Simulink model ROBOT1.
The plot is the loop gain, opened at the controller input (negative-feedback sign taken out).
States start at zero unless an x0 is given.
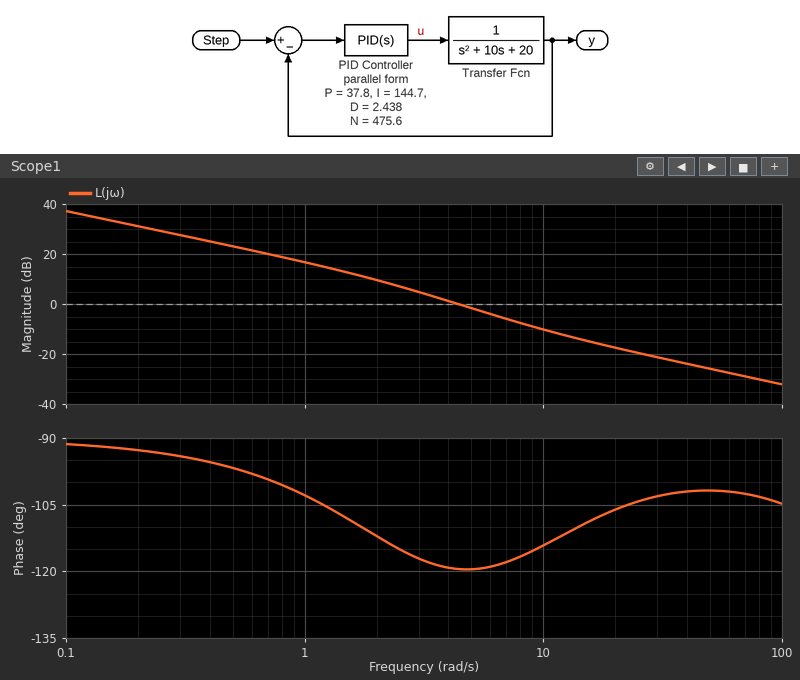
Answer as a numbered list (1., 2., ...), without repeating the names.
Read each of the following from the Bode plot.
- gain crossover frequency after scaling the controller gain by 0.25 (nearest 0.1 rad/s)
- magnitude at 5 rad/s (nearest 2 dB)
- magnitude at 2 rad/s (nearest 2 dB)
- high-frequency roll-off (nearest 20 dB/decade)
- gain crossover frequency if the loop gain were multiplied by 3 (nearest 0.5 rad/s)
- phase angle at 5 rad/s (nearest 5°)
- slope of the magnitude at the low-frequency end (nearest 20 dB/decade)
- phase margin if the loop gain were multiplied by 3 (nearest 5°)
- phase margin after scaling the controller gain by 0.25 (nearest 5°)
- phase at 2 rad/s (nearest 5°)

1. 1.6 rad/s
2. -2 dB
3. 10 dB
4. -20 dB/decade
5. 9.5 rad/s
6. -120°
7. -20 dB/decade
8. 65°
9. 70°
10. -110°
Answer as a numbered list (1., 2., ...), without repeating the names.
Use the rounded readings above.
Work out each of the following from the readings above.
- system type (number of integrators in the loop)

1. 1
